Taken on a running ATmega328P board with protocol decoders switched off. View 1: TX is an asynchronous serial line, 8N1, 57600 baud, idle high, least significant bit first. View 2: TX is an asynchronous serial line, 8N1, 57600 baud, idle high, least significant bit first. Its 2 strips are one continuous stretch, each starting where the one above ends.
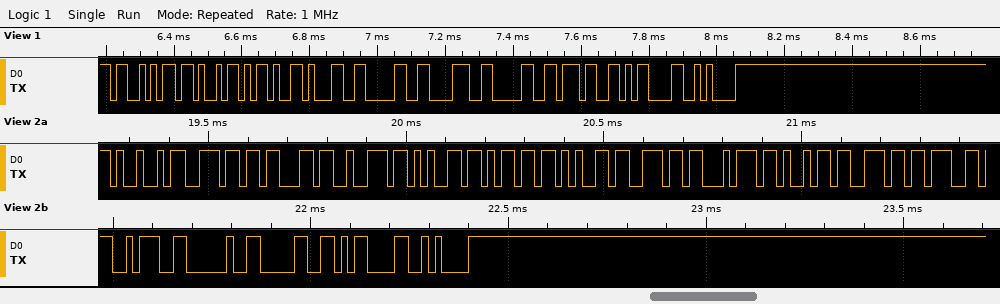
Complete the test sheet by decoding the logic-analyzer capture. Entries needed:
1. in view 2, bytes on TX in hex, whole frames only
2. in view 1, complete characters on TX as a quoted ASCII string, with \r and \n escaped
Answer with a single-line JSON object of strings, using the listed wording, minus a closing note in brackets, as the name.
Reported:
{"in view 2, bytes on TX in hex, whole frames only": "0x49 0x6E 0x63 0x72 0x65 0x6D 0x65 0x6E 0x74 0x69 0x6E 0x67 0x3A 0x20 0x30 0x0D 0x0A", "in view 1, complete characters on TX as a quoted ASCII string, with \\r and \\n escaped": "\"SK-10807\\r\\n\""}
